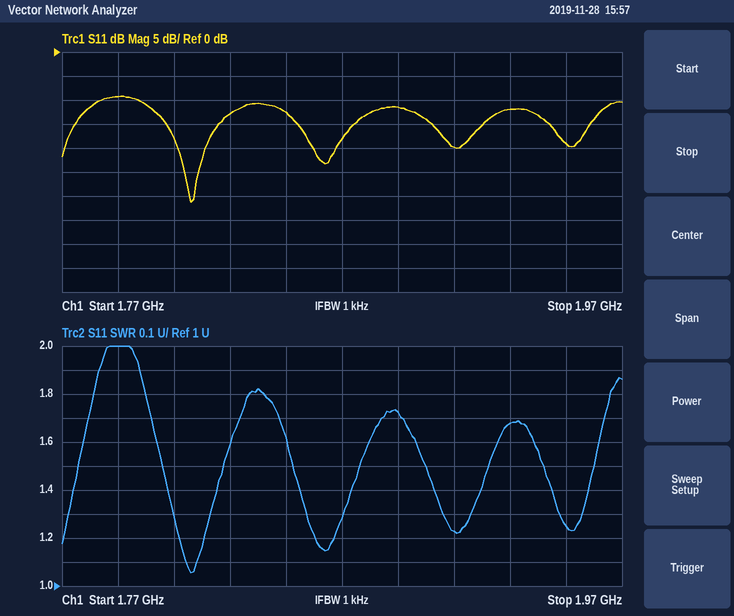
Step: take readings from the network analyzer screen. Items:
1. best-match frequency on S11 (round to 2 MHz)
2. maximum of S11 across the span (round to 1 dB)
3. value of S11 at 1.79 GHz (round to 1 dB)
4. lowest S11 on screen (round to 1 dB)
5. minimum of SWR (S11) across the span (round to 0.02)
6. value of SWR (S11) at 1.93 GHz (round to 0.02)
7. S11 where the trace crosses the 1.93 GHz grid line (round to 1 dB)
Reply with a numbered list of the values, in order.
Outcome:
1. 1.816 GHz
2. -9 dB
3. -9 dB
4. -31 dB
5. 1.06
6. 1.68
7. -12 dB
